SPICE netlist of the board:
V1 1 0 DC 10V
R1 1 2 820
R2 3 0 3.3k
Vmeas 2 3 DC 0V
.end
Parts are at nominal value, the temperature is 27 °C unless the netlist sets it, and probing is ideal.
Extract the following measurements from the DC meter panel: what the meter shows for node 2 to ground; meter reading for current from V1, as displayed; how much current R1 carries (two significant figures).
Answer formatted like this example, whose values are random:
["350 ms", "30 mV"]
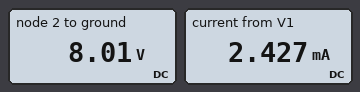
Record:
["8.01 V", "2.427 mA", "2.4 mA"]
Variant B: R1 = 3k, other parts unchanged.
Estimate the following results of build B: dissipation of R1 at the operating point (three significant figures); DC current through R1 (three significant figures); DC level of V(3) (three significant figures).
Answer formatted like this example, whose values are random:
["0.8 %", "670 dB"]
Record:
["7.56 mW", "1.59 mA", "5.24 V"]
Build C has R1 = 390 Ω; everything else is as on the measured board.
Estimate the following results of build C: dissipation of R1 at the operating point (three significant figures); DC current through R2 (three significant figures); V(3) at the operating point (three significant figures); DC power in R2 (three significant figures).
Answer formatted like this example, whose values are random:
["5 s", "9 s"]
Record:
["2.86 mW", "2.71 mA", "8.94 V", "24.2 mW"]
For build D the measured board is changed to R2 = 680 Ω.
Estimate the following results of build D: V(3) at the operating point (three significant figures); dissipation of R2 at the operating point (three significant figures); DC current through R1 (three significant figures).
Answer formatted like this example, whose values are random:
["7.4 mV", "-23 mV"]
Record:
["4.53 V", "30.2 mW", "6.67 mA"]
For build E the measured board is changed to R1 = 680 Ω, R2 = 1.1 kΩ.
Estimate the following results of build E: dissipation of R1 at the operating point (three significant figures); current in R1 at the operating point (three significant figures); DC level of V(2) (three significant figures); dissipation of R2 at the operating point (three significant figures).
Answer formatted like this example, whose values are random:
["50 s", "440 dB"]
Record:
["21.5 mW", "5.62 mA", "6.18 V", "34.7 mW"]
